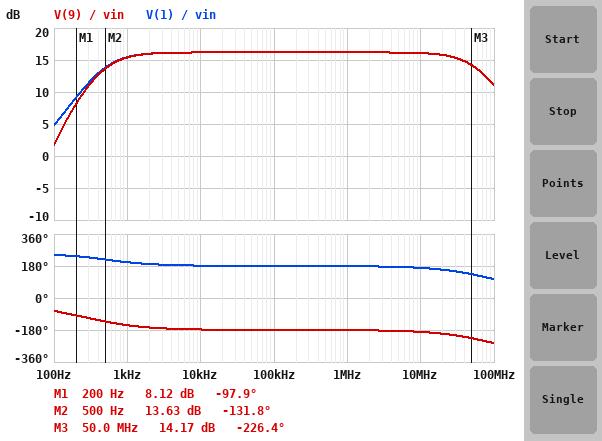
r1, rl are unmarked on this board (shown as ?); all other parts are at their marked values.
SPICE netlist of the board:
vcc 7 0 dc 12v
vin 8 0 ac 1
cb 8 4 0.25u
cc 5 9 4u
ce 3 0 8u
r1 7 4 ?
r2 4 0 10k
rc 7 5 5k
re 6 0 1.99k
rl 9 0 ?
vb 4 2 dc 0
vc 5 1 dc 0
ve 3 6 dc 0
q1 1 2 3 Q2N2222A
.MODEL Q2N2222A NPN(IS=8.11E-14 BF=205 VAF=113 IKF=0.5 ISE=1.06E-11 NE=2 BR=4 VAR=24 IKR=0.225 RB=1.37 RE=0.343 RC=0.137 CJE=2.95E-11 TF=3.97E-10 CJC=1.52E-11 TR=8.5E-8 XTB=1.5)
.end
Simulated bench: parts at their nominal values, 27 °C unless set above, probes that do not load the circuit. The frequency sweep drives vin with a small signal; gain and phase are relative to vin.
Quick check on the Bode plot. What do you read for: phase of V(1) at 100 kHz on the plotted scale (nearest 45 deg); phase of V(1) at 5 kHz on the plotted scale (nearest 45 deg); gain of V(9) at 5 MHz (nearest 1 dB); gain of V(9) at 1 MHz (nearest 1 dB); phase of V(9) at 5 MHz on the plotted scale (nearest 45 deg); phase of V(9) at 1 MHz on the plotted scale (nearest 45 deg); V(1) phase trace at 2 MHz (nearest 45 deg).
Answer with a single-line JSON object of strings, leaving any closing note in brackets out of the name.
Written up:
{"phase of V(1) at 100 kHz on the plotted scale": "180 deg", "phase of V(1) at 5 kHz on the plotted scale": "180 deg", "gain of V(9) at 5 MHz": "16 dB", "gain of V(9) at 1 MHz": "16 dB", "phase of V(9) at 5 MHz on the plotted scale": "-180 deg", "phase of V(9) at 1 MHz on the plotted scale": "-180 deg", "V(1) phase trace at 2 MHz": "180 deg"}
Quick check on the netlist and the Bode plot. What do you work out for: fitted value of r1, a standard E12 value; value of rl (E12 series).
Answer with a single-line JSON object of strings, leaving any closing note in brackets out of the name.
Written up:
{"fitted value of r1, a standard E12 value": "68 kΩ", "value of rl": "390 Ω"}
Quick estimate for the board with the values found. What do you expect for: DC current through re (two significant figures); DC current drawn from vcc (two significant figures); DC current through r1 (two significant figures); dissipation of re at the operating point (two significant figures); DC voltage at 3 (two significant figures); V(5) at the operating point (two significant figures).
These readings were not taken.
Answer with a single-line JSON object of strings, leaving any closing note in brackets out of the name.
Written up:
{"DC current through re": "470 µA", "DC current drawn from vcc": "620 µA", "DC current through r1": "150 µA", "dissipation of re at the operating point": "440 µW", "DC voltage at 3": "930 mV", "V(5) at the operating point": "9.7 V"}
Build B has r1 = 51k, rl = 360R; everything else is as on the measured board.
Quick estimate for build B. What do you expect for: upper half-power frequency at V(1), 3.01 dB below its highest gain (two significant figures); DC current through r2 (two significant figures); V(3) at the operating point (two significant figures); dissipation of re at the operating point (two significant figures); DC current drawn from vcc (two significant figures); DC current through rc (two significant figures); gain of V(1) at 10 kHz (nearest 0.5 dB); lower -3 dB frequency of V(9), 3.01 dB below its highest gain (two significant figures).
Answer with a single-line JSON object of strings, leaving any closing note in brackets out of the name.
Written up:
{"upper half-power frequency at V(1), 3.01 dB below its highest gain": "65 MHz", "DC current through r2": "190 µA", "V(3) at the operating point": "1.3 V", "dissipation of re at the operating point": "910 µW", "DC current drawn from vcc": "870 µA", "DC current through rc": "670 µA", "gain of V(1) at 10 kHz": "18.5 dB", "lower -3 dB frequency of V(9), 3.01 dB below its highest gain": "630 Hz"}
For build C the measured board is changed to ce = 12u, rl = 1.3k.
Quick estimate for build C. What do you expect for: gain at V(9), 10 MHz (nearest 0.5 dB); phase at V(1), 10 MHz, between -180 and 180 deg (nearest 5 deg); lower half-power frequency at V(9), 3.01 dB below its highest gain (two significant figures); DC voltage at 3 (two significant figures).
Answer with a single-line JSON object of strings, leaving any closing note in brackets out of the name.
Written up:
{"gain at V(9), 10 MHz": "24.5 dB", "phase at V(1), 10 MHz, between -180 and 180 deg": "155 deg", "lower half-power frequency at V(9), 3.01 dB below its highest gain": "330 Hz", "DC voltage at 3": "930 mV"}
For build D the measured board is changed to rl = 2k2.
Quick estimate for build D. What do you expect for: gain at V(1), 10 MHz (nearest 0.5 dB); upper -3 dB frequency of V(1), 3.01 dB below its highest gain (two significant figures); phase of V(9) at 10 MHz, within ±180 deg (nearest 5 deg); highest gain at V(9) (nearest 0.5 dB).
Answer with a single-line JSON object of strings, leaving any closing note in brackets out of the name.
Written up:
{"gain at V(1), 10 MHz": "27.0 dB", "upper -3 dB frequency of V(1), 3.01 dB below its highest gain": "15 MHz", "phase of V(9) at 10 MHz, within ±180 deg": "145 deg", "highest gain at V(9)": "28.5 dB"}
